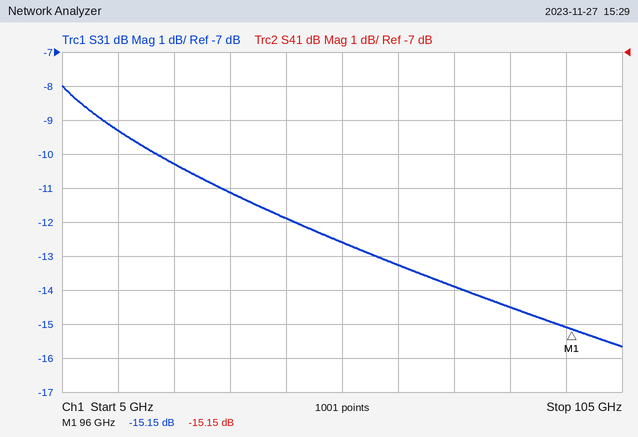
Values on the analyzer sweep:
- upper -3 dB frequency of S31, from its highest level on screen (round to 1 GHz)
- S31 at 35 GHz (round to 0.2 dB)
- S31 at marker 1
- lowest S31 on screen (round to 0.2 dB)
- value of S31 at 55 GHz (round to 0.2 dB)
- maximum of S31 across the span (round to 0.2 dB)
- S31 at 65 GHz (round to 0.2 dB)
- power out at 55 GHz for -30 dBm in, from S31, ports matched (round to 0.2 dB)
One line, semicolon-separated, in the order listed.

33 GHz; -11.2 dB; -15.15 dB; -15.6 dB; -12.6 dB; -8.0 dB; -13.2 dB; -42.6 dBm
